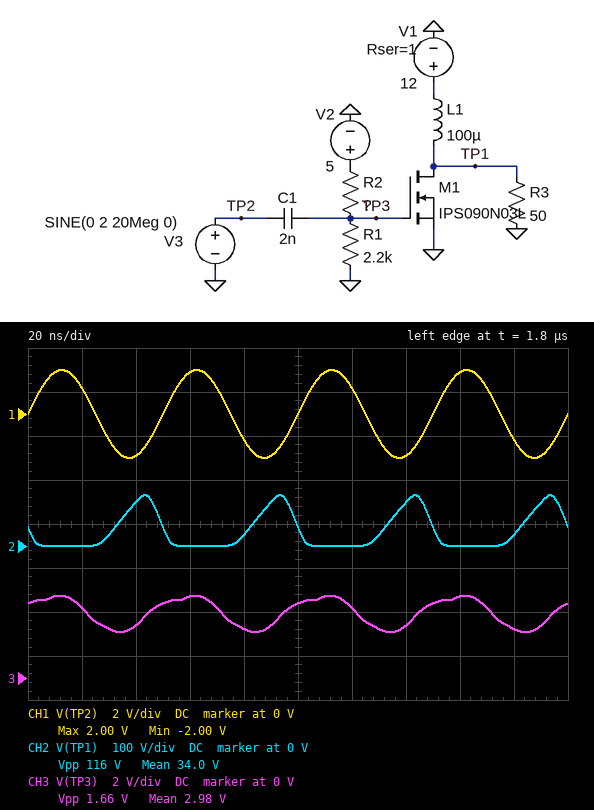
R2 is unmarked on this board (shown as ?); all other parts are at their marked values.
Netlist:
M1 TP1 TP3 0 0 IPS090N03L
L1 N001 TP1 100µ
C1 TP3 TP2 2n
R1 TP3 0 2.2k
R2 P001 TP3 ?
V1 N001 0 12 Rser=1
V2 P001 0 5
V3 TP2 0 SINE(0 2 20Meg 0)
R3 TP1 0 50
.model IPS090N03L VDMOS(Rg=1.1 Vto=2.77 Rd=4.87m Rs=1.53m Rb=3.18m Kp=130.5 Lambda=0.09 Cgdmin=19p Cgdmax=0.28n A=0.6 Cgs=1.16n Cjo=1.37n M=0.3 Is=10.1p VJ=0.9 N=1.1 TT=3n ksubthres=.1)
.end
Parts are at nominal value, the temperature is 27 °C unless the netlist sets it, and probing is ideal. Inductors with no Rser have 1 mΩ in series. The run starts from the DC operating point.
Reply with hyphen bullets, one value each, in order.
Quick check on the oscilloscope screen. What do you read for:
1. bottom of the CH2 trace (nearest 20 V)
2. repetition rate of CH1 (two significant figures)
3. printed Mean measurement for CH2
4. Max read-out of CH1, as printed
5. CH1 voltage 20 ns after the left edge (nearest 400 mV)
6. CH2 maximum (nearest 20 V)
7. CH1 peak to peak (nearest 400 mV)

- 0 V
- 20 MHz
- 34.0 V
- 2.00 V
- 1.2 V
- 120 V
- 4.0 V
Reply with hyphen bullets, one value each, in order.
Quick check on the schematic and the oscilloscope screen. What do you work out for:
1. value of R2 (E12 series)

- 1.5 kΩ
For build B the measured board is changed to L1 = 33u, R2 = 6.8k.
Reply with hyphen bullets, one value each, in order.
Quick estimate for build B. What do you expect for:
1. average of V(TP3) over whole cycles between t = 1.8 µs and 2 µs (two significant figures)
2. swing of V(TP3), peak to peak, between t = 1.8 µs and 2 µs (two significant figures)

- 1.2 V
- 2.5 V
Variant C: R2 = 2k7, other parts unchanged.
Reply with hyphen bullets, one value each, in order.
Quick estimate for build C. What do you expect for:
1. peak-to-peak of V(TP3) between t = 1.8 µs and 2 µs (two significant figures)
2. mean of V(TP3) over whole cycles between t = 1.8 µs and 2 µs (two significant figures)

- 2.3 V
- 2.1 V
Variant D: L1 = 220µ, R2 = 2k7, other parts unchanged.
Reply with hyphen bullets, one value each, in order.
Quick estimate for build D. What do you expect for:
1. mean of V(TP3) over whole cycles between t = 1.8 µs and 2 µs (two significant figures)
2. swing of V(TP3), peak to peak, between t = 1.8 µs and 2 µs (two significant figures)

- 2.1 V
- 2.3 V
